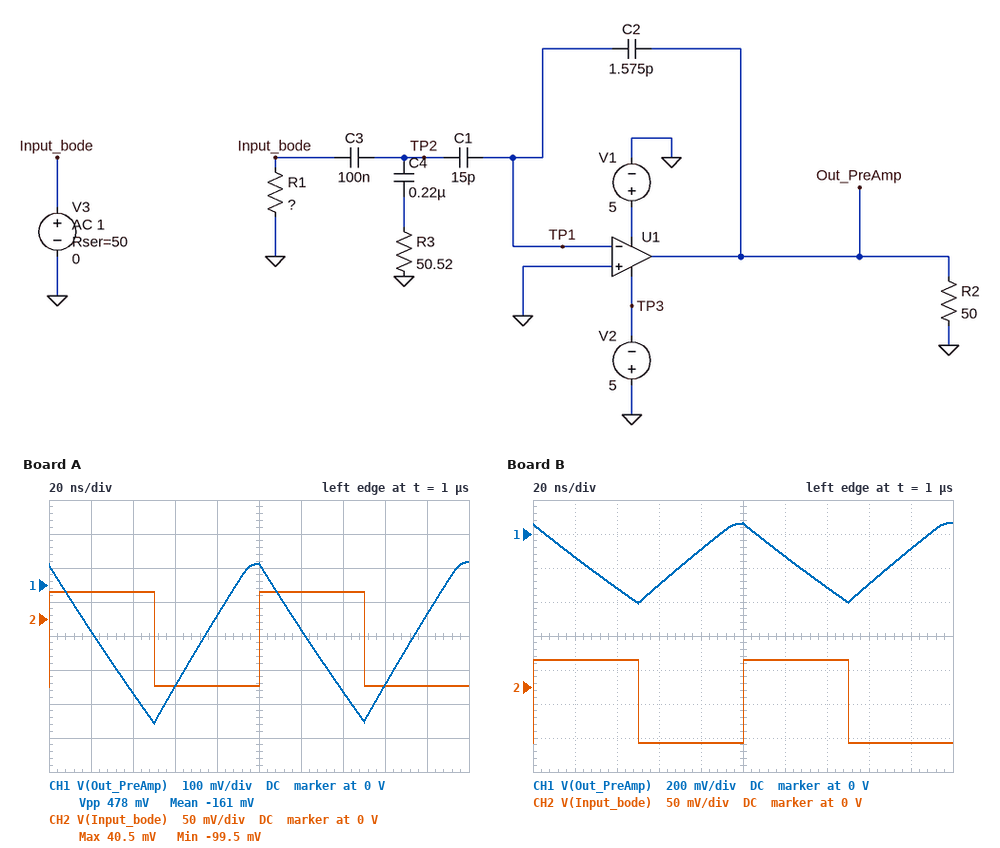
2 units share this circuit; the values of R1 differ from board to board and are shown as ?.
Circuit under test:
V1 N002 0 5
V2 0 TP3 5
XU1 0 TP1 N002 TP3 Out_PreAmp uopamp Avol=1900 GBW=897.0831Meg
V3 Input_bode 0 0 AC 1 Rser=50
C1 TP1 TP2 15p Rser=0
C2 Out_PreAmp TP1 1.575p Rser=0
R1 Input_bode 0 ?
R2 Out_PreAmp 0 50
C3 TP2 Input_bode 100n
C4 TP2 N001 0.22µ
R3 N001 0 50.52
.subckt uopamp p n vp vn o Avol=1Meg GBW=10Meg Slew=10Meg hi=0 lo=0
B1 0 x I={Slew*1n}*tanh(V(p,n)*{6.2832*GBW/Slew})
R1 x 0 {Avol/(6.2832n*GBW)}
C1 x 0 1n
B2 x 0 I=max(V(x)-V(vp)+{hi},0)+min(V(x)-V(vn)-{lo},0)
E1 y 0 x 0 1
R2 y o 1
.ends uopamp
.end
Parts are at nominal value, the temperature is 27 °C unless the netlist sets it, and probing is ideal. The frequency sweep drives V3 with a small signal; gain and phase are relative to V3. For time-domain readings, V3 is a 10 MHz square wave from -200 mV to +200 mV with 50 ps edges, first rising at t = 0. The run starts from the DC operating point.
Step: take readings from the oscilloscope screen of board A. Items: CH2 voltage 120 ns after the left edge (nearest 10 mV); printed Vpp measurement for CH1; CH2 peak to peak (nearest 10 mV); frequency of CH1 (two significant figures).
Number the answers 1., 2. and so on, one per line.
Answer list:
1. 40 mV
2. 478 mV
3. 140 mV
4. 10 MHz
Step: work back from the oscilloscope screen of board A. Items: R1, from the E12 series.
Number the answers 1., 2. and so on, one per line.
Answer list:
1. 56 Ω
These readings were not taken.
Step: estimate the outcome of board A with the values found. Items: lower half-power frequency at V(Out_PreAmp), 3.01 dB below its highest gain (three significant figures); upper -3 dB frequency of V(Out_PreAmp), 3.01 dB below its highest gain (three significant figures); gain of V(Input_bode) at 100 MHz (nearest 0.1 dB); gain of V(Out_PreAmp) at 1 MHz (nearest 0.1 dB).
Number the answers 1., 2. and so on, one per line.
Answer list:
1. 22.2 kHz
2. 74.8 MHz
3. -9.8 dB
4. 10.3 dB
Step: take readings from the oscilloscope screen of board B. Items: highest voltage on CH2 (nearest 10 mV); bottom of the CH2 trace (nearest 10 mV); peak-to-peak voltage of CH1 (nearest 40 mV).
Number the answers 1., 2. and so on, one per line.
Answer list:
1. 40 mV
2. -80 mV
3. 480 mV
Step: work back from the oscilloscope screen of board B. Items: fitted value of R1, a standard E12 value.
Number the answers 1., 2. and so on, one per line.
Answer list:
1. 39 Ω
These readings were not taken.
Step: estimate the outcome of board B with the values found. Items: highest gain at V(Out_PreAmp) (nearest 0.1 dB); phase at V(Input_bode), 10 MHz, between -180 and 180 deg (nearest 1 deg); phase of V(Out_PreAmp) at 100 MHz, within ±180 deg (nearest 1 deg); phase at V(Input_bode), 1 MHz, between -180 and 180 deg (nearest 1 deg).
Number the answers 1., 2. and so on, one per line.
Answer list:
1. 9.2 dB
2. -1 deg
3. 126 deg
4. -1 deg
